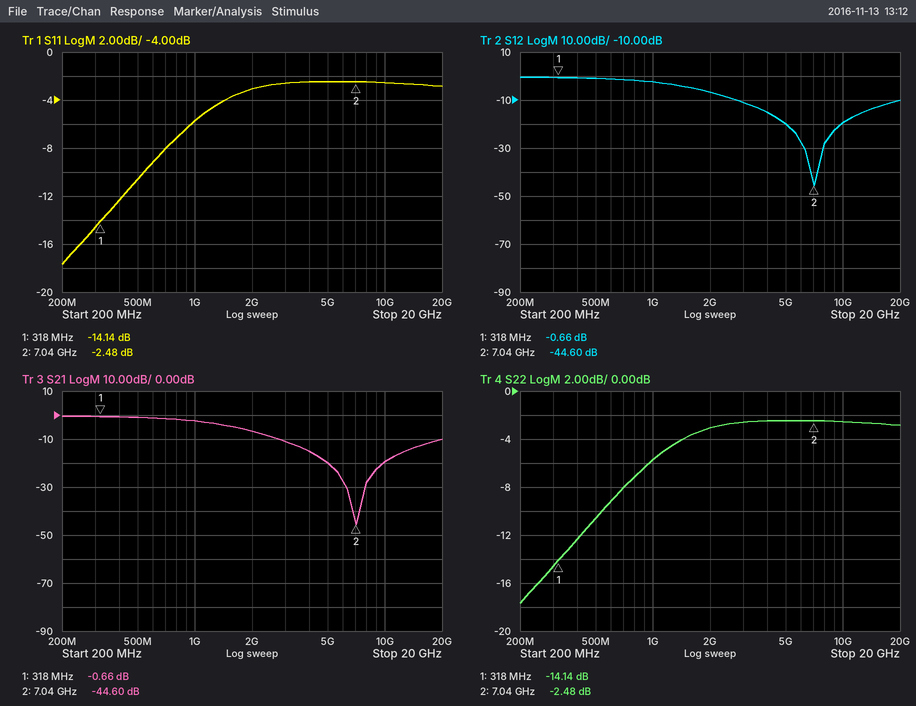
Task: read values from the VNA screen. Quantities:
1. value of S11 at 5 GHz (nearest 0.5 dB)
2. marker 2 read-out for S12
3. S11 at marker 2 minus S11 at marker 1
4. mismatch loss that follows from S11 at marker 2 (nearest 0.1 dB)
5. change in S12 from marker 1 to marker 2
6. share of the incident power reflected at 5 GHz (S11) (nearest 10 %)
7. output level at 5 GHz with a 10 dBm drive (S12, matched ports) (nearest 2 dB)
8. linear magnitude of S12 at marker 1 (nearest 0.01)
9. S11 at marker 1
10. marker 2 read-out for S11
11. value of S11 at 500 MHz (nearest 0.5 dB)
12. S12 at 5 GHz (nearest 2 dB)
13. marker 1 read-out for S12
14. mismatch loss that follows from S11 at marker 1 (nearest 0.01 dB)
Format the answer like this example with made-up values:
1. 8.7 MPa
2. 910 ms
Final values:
1. -2.5 dB
2. -44.60 dB
3. 11.66 dB
4. 3.6 dB
5. -43.94 dB
6. 60 %
7. -10 dBm
8. 0.93
9. -14.14 dB
10. -2.48 dB
11. -10.5 dB
12. -20 dB
13. -0.66 dB
14. 0.17 dB
